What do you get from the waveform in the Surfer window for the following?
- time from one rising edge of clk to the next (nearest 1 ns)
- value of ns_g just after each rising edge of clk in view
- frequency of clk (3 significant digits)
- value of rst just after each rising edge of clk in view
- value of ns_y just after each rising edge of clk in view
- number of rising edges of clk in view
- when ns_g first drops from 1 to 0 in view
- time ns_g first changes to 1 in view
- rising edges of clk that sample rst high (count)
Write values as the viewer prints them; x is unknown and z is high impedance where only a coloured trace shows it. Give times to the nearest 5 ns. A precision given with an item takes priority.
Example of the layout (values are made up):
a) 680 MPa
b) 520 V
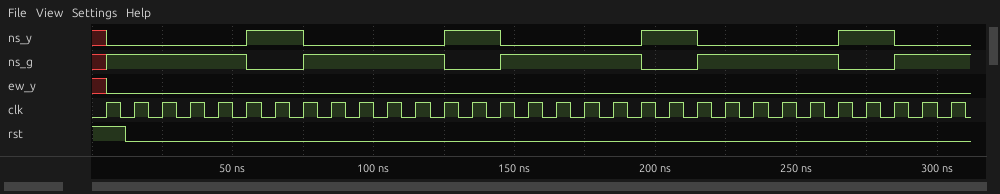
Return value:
a) 10 ns
b) 1 1 1 1 1 0 0 1 1 1 1 1 0 0 1 1 1 1 1 0 0 1 1 1 1 1 0 0 1 1 1
c) 100 MHz
d) 1 0 0 0 0 0 0 0 0 0 0 0 0 0 0 0 0 0 0 0 0 0 0 0 0 0 0 0 0 0 0
e) 0 0 0 0 0 1 1 0 0 0 0 0 1 1 0 0 0 0 0 1 1 0 0 0 0 0 1 1 0 0 0
f) 31
g) 55 ns
h) 5 ns
i) 1
